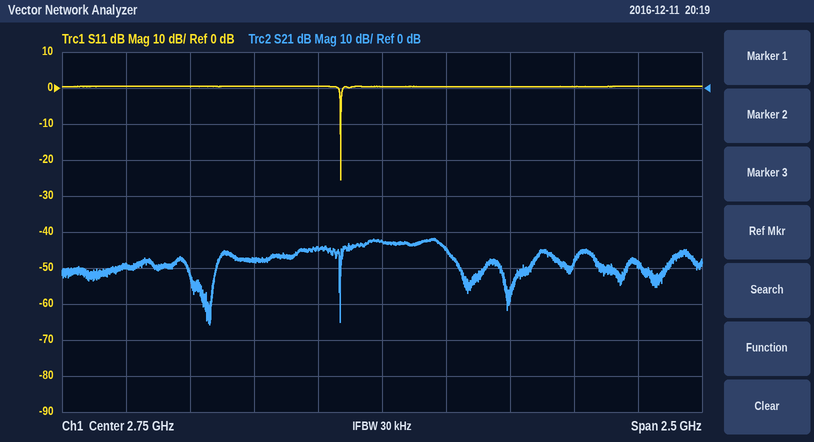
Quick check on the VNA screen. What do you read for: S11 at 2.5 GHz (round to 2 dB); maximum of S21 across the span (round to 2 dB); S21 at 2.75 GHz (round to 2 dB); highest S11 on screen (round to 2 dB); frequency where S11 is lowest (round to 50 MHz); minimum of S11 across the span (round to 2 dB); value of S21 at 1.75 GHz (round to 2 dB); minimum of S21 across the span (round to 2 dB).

0 dB
-42 dB
-42 dB
0 dB
2.60 GHz
-26 dB
-50 dB
-66 dB
